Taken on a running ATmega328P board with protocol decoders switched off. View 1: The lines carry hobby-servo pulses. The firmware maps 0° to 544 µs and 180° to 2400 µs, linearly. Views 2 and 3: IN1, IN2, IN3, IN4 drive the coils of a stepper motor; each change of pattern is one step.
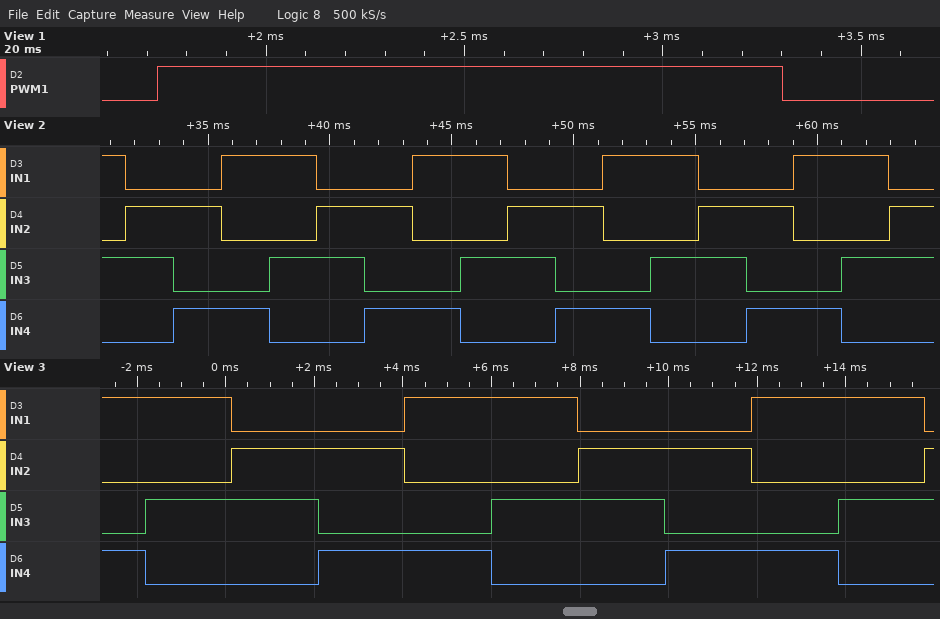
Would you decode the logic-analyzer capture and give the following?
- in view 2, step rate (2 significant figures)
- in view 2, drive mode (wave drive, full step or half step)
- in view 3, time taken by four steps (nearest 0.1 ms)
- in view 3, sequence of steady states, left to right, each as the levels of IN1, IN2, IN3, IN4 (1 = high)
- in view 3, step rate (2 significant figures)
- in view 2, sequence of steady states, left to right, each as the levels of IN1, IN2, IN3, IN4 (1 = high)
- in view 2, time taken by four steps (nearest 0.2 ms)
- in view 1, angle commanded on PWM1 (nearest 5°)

510 steps/s
full step
7.8 ms
1001 1010 0110 0101 1001 1010 0110 0101 1001 1010 0110
510 steps/s
1010 0110 0101 1001 1010 0110 0101 1001 1010 0110 0101 1001 1010 0110 0101 1001 1010 0110
7.8 ms
100°
